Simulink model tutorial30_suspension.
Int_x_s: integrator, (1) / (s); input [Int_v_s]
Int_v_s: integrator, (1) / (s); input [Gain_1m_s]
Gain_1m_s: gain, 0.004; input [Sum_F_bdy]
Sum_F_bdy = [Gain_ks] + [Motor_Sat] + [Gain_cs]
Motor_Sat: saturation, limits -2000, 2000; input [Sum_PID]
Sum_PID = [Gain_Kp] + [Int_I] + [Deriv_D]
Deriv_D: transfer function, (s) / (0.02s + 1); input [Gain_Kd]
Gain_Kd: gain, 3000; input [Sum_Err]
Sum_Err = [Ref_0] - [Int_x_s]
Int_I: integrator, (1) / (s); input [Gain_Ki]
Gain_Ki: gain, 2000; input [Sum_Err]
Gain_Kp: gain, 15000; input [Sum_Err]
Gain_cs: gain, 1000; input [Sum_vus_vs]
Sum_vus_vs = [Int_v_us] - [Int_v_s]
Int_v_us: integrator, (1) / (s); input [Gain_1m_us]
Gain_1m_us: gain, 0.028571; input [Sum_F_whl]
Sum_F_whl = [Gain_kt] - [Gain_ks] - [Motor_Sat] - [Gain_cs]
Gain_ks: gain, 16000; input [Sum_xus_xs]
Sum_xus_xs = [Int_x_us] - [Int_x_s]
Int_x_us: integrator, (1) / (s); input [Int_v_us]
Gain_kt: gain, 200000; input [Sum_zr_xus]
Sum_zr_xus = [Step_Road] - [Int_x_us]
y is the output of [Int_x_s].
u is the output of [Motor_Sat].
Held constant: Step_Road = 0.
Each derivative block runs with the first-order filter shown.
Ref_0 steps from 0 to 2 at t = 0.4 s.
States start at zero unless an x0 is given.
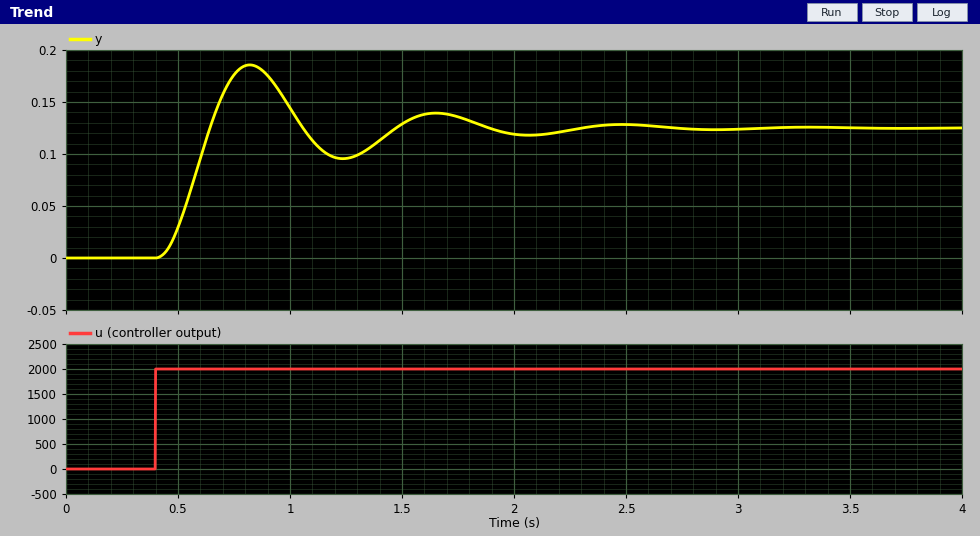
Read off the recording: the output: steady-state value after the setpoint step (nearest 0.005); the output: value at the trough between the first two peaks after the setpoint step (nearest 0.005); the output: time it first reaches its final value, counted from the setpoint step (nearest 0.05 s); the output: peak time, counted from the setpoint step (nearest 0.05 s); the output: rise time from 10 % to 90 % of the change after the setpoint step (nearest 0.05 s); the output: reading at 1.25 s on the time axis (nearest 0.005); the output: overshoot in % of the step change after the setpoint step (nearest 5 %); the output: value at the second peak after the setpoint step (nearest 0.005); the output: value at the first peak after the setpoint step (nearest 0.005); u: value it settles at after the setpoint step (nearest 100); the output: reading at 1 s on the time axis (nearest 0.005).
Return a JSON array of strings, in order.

["0.125", "0.095", "0.25 s", "0.40 s", "0.15 s", "0.095", "50 %", "0.140", "0.185", "2000", "0.145"]
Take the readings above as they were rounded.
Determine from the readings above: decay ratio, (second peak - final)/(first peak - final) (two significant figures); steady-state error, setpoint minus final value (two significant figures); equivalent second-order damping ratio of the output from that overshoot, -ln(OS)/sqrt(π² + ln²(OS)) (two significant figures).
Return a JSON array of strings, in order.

["0.25", "1.9", "0.22"]
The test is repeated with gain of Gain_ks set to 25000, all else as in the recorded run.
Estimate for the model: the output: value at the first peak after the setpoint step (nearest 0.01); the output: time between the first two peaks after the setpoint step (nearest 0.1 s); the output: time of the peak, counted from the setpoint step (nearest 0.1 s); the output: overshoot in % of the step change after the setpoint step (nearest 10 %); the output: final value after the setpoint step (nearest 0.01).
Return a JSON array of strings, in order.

["0.13", "0.7 s", "0.3 s", "60 %", "0.08"]
